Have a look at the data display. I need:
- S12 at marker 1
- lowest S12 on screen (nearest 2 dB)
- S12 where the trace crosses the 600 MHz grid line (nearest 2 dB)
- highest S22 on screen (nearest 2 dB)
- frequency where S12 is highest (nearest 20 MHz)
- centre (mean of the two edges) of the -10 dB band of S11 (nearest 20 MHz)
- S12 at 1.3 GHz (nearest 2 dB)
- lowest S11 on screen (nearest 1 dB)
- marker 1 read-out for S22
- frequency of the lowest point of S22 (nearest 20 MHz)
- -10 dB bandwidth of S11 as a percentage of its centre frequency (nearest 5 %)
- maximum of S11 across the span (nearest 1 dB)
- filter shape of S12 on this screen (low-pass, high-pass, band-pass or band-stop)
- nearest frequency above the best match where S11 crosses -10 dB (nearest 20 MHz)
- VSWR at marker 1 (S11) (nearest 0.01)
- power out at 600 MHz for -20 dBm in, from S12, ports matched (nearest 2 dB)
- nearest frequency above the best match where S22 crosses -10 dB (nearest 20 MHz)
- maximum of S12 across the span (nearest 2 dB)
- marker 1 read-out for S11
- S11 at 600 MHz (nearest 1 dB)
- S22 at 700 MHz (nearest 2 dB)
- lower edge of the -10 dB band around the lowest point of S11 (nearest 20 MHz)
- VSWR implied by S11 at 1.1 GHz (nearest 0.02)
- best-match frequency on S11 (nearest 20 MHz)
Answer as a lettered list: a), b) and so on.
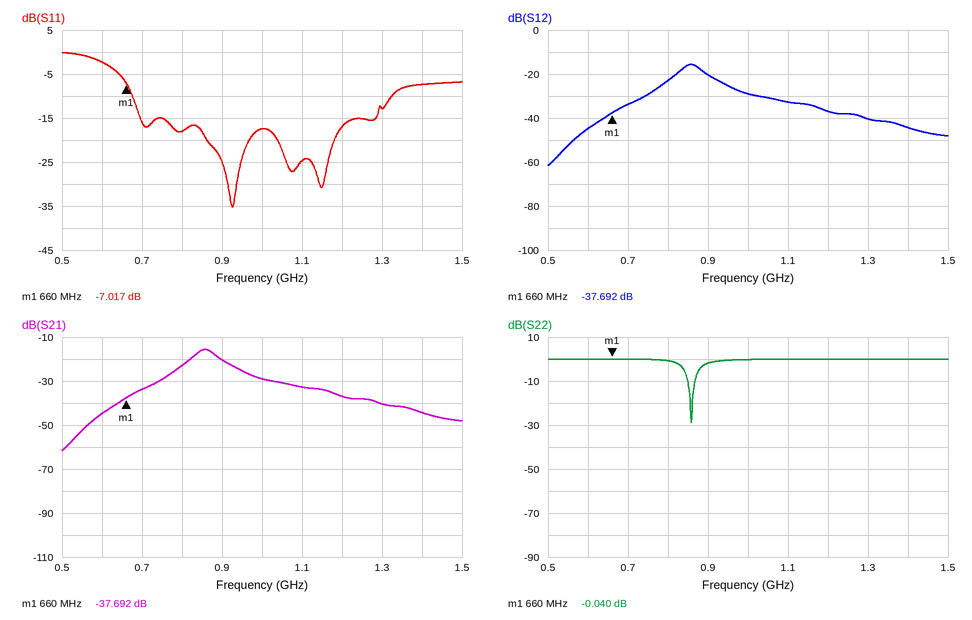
a) -37.692 dB
b) -62 dB
c) -44 dB
d) 0 dB
e) 860 MHz
f) 1.00 GHz
g) -40 dB
h) -35 dB
i) -0.040 dB
j) 860 MHz
k) 65 %
l) 0 dB
m) band-pass
n) 1.32 GHz
o) 2.61
p) -64 dBm
q) 860 MHz
r) -16 dB
s) -7.017 dB
t) -2 dB
u) 0 dB
v) 680 MHz
w) 1.12
x) 920 MHz
